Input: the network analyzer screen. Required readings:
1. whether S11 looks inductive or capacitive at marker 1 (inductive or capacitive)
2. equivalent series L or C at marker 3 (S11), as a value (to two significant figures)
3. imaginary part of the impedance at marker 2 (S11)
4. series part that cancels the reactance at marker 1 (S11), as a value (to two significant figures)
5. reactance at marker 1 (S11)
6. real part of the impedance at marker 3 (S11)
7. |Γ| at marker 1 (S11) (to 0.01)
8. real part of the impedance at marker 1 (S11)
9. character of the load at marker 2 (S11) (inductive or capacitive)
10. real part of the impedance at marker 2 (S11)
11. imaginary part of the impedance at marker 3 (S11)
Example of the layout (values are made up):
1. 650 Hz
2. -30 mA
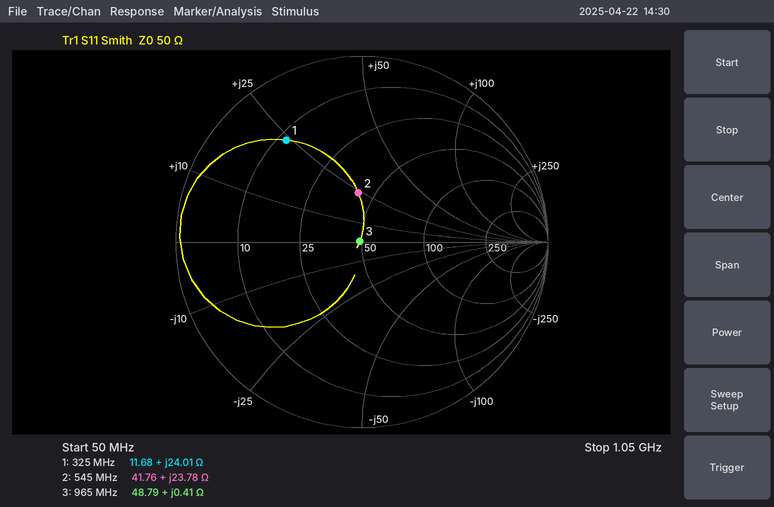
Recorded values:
1. inductive
2. 68 pH
3. +23.78 Ω
4. 20 pF
5. +24.01 Ω
6. 48.79 Ω
7. 0.68
8. 11.68 Ω
9. inductive
10. 41.76 Ω
11. +0.41 Ω
